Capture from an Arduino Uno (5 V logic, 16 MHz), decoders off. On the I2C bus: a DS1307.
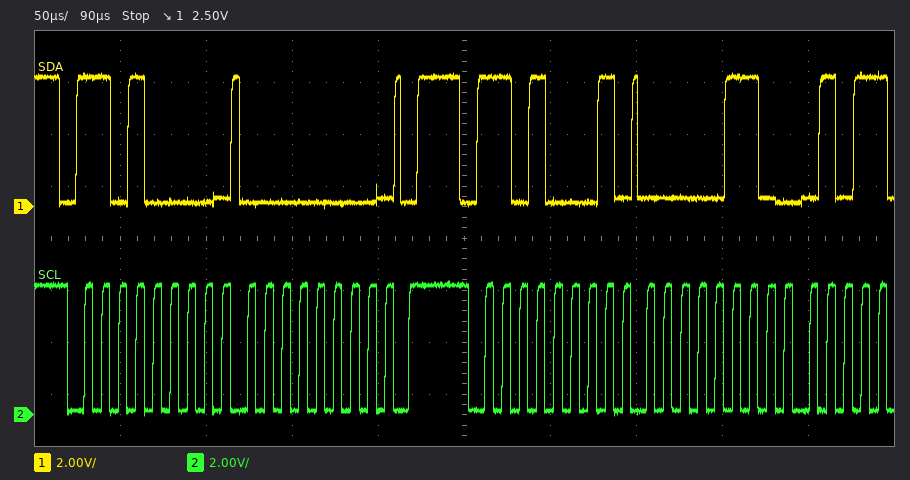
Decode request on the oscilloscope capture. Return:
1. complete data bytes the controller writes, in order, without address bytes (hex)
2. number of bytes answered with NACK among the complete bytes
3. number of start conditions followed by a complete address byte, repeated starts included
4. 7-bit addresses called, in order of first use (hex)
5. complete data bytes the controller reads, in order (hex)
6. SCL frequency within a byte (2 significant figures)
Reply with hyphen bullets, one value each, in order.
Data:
- 00
- 0
- 2
- 0x68
- 06
- 100 kHz
